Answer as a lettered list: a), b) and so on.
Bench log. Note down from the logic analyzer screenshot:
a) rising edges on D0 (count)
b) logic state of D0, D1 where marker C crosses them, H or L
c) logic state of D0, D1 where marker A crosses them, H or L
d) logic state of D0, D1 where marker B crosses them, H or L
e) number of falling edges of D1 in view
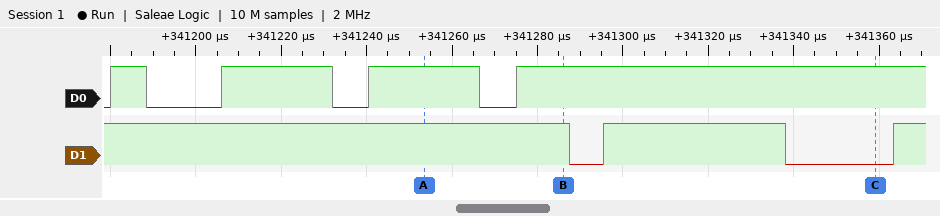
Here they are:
a) 4
b) D0=H, D1=L
c) D0=H, D1=H
d) D0=H, D1=H
e) 2
